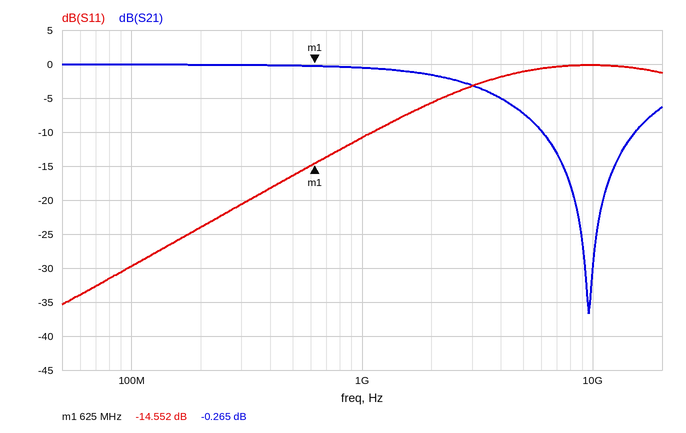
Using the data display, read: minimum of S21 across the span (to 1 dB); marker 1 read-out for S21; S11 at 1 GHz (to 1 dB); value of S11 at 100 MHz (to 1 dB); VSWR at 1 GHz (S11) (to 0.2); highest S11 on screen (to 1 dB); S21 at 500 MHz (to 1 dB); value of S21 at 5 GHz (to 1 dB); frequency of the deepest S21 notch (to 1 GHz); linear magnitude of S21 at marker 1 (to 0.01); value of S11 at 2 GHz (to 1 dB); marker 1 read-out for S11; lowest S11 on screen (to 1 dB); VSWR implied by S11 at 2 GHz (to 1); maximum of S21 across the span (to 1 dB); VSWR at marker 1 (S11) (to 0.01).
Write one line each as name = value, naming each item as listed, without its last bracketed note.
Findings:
minimum of S21 across the span = -37 dB
marker 1 read-out for S21 = -0.265 dB
S11 at 1 GHz = -11 dB
value of S11 at 100 MHz = -30 dB
VSWR at 1 GHz (S11) = 1.8
highest S11 on screen = 0 dB
S21 at 500 MHz = 0 dB
value of S21 at 5 GHz = -7 dB
frequency of the deepest S21 notch = 10 GHz
linear magnitude of S21 at marker 1 = 0.97
value of S11 at 2 GHz = -6 dB
marker 1 read-out for S11 = -14.552 dB
lowest S11 on screen = -35 dB
VSWR implied by S11 at 2 GHz = 3
maximum of S21 across the span = 0 dB
VSWR at marker 1 (S11) = 1.46
